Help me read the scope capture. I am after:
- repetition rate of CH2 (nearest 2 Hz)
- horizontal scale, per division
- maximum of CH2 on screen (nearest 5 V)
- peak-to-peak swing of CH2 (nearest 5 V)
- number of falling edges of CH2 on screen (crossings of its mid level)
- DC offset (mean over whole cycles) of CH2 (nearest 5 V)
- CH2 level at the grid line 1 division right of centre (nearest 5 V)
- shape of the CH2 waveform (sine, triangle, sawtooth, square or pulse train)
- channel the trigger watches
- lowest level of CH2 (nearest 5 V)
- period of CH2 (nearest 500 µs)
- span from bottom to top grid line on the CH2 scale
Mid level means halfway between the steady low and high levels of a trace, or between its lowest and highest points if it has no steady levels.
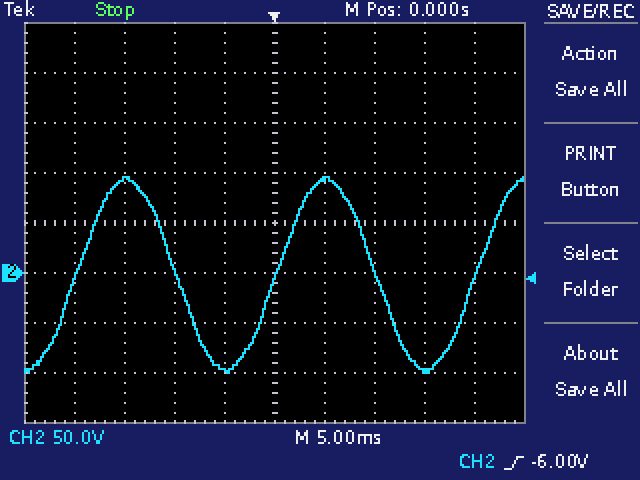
50 Hz
5 ms
95 V
195 V
2
0 V
95 V
sine
CH2
-100 V
20.0 ms
400 V
